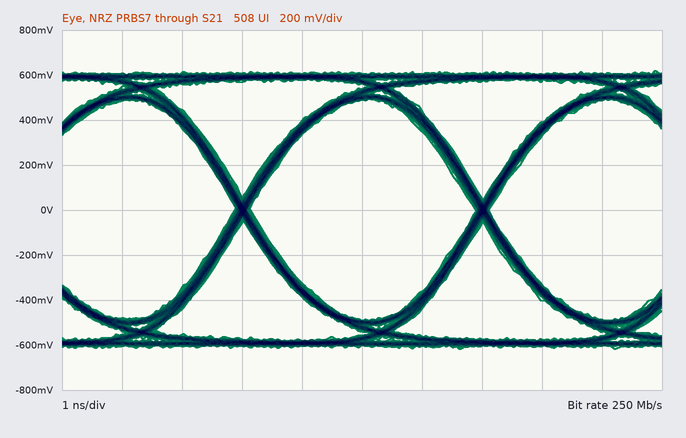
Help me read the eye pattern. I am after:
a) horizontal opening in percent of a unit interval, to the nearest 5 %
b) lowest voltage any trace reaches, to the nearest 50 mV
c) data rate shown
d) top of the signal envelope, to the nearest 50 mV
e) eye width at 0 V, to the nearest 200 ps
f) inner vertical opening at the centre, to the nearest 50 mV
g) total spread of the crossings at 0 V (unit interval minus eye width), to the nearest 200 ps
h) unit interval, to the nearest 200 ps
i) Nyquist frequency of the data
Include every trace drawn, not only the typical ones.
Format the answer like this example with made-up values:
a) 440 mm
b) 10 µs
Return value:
a) 95 %
b) -600 mV
c) 250 Mb/s
d) 600 mV
e) 3.8 ns
f) 1.00 V
g) 200 ps
h) 4.0 ns
i) 125 MHz
